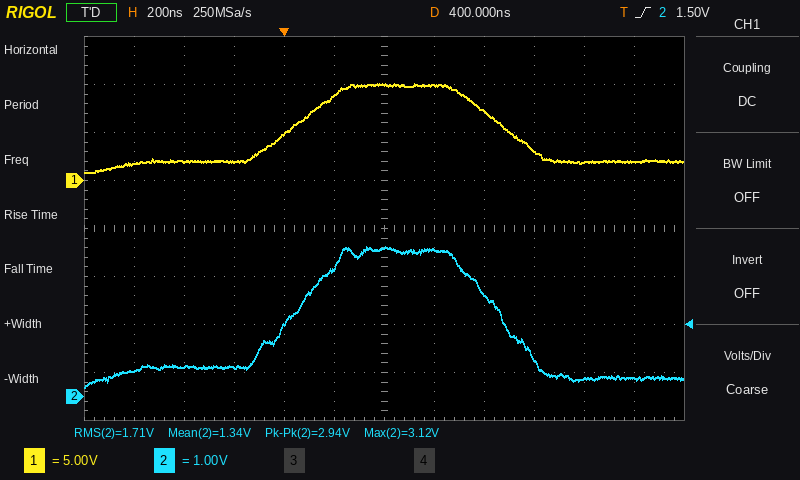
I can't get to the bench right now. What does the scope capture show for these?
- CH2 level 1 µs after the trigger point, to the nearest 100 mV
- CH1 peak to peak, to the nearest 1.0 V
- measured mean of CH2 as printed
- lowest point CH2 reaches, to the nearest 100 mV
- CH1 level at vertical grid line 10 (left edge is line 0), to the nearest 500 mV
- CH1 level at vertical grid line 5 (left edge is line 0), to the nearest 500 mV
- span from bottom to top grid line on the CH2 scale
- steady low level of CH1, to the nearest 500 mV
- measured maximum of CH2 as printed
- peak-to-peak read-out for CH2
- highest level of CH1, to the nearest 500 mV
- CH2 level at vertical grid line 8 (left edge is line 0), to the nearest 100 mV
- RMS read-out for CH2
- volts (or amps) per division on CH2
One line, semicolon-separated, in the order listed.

800 mV; 9.0 V; 1.34 V; 200 mV; 2.0 V; 9.0 V; 8 V; 2.0 V; 3.12 V; 2.94 V; 10.0 V; 2.1 V; 1.71 V; 1 V
